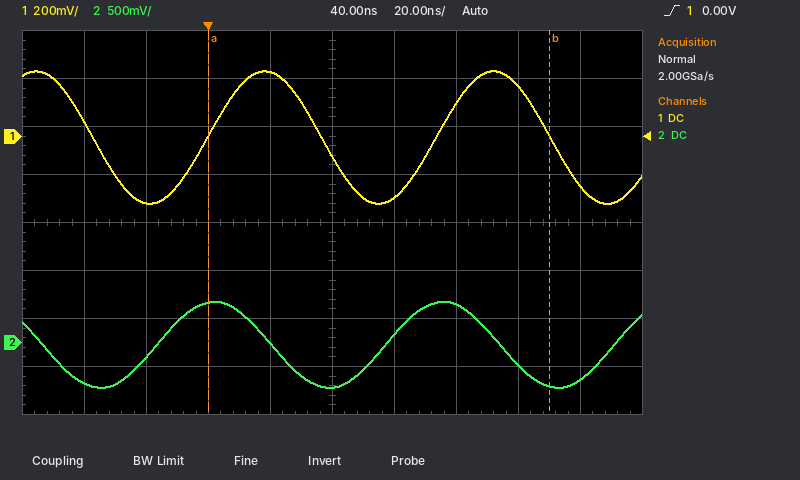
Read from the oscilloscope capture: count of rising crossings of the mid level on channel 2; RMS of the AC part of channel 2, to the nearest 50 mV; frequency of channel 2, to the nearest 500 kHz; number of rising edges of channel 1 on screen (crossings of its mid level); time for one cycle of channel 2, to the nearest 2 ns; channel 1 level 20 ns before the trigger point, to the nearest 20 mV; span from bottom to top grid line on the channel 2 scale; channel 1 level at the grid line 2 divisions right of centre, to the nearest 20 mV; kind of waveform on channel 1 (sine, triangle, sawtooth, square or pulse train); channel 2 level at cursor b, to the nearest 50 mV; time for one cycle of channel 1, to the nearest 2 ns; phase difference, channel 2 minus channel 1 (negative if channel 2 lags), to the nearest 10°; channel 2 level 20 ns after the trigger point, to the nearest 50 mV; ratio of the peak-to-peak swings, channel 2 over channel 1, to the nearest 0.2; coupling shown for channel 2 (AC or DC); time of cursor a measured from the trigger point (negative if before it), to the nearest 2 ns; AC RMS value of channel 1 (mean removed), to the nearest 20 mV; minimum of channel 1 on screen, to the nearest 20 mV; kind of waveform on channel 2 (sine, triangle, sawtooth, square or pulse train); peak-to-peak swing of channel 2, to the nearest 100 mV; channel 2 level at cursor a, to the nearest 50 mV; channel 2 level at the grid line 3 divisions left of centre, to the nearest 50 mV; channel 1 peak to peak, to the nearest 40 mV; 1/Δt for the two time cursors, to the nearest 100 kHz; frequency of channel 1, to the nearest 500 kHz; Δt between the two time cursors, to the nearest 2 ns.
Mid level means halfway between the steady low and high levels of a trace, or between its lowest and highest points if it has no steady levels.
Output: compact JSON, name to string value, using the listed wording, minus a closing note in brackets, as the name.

{"count of rising crossings of the mid level on channel 2": "3", "RMS of the AC part of channel 2, to the nearest 50 mV": "300 mV", "frequency of channel 2, to the nearest 500 kHz": "13.5 MHz", "number of rising edges of channel 1 on screen": "2", "time for one cycle of channel 2, to the nearest 2 ns": "74 ns", "channel 1 level 20 ns before the trigger point, to the nearest 20 mV": "-280 mV", "span from bottom to top grid line on the channel 2 scale": "4 V", "channel 1 level at the grid line 2 divisions right of centre, to the nearest 20 mV": "140 mV", "kind of waveform on channel 1": "sine", "channel 2 level at cursor b, to the nearest 50 mV": "-450 mV", "time for one cycle of channel 1, to the nearest 2 ns": "74 ns", "phase difference, channel 2 minus channel 1 (negative if channel 2 lags), to the nearest 10°": "+80°", "channel 2 level 20 ns after the trigger point, to the nearest 50 mV": "0 mV", "ratio of the peak-to-peak swings, channel 2 over channel 1, to the nearest 0.2": "1.6", "coupling shown for channel 2": "DC", "time of cursor a measured from the trigger point (negative if before it), to the nearest 2 ns": "0 ns", "AC RMS value of channel 1 (mean removed), to the nearest 20 mV": "200 mV", "minimum of channel 1 on screen, to the nearest 20 mV": "-280 mV", "kind of waveform on channel 2": "sine", "peak-to-peak swing of channel 2, to the nearest 100 mV": "900 mV", "channel 2 level at cursor a, to the nearest 50 mV": "400 mV", "channel 2 level at the grid line 3 divisions left of centre, to the nearest 50 mV": "-150 mV", "channel 1 peak to peak, to the nearest 40 mV": "560 mV", "1/Δt for the two time cursors, to the nearest 100 kHz": "9.1 MHz", "frequency of channel 1, to the nearest 500 kHz": "13.5 MHz", "Δt between the two time cursors, to the nearest 2 ns": "110 ns"}
